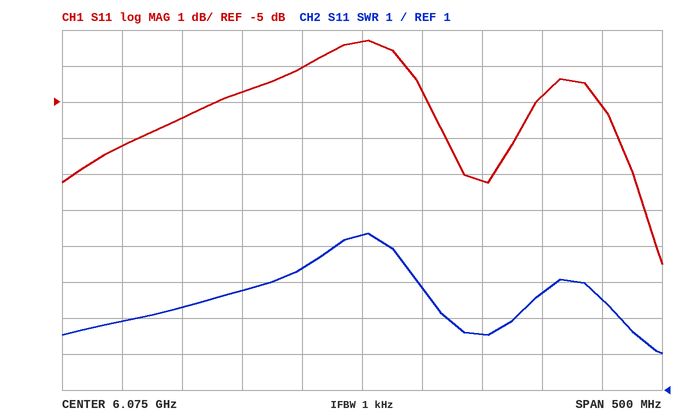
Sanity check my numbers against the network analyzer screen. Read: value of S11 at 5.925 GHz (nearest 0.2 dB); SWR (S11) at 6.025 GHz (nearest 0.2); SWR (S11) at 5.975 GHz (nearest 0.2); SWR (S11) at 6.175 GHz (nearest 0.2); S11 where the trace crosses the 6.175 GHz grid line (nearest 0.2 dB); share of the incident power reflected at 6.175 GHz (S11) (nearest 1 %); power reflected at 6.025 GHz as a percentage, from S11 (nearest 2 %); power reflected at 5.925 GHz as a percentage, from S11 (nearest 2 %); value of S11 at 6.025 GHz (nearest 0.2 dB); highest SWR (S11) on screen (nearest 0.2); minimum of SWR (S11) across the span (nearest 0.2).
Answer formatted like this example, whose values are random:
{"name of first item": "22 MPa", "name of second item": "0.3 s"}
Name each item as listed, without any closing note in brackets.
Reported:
{"value of S11 at 5.925 GHz": "-5.4 dB", "SWR (S11) at 6.025 GHz": "4.4", "SWR (S11) at 5.975 GHz": "3.8", "SWR (S11) at 6.175 GHz": "2.6", "S11 where the trace crosses the 6.175 GHz grid line": "-7.2 dB", "share of the incident power reflected at 6.175 GHz (S11)": "19 %", "power reflected at 6.025 GHz as a percentage, from S11": "40 %", "power reflected at 5.925 GHz as a percentage, from S11": "28 %", "value of S11 at 6.025 GHz": "-4.0 dB", "highest SWR (S11) on screen": "5.4", "minimum of SWR (S11) across the span": "2.0"}
